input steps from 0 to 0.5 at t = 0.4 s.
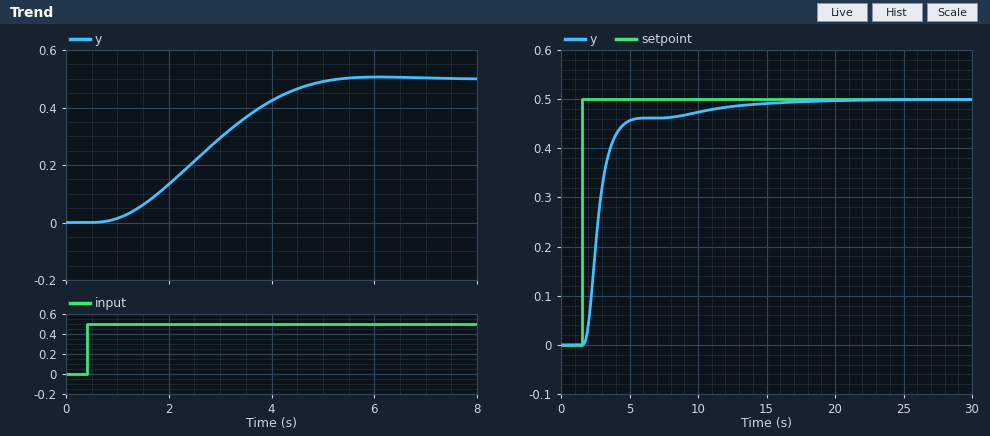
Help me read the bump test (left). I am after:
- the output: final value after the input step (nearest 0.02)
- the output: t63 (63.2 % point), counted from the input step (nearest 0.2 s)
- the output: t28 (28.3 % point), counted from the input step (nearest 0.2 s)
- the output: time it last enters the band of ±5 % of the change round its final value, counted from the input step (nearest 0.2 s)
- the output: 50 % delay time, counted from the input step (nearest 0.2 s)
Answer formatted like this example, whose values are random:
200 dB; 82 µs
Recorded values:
0.50; 2.8 s; 1.6 s; 4.2 s; 2.4 s
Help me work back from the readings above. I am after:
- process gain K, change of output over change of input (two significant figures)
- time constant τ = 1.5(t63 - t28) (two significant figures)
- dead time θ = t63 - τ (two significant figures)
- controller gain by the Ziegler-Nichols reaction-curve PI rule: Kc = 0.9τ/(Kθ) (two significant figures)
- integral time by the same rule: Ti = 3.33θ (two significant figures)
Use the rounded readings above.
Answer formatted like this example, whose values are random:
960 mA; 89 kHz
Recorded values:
1.0; 1.8 s; 1.0 s; 1.6; 3.3 s
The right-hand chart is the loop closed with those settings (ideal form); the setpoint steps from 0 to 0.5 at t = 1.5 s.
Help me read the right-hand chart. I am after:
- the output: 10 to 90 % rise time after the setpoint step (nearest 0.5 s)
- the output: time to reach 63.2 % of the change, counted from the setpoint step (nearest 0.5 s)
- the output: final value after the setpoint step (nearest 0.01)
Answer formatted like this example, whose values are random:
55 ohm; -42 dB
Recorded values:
2.5 s; 1.5 s; 0.50
